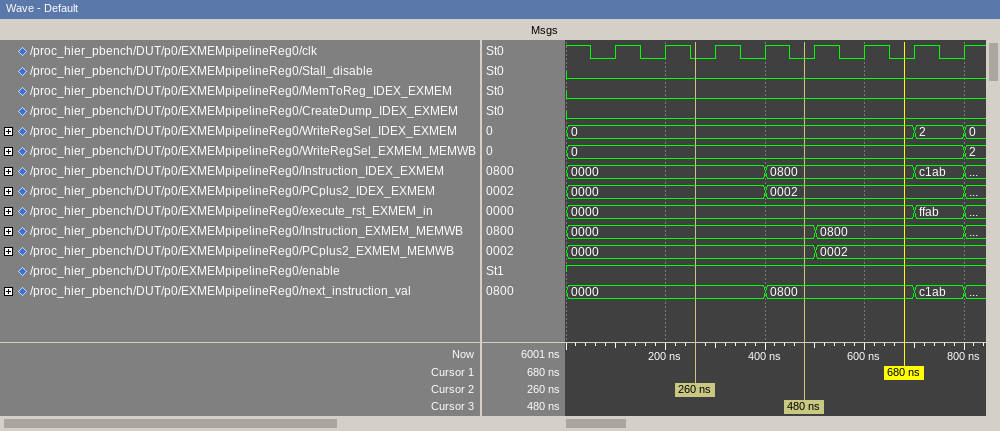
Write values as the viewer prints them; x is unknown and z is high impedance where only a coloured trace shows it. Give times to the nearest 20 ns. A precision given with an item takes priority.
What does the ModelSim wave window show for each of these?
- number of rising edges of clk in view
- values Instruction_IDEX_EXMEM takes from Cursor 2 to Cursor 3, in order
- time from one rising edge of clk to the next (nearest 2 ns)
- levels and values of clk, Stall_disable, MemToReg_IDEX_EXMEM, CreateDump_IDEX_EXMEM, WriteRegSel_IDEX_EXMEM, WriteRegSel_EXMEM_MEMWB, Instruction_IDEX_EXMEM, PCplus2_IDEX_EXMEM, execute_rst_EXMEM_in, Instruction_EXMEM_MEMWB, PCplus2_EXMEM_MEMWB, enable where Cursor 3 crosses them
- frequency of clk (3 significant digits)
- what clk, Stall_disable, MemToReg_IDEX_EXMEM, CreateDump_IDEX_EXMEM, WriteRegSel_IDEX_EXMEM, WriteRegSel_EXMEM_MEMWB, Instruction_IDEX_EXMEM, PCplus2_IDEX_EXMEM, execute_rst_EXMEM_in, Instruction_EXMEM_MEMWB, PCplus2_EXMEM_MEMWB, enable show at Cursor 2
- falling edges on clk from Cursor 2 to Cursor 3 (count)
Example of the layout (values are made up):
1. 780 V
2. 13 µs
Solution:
1. 8
2. 0000, 0800
3. 100 ns
4. clk=0, Stall_disable=0, MemToReg_IDEX_EXMEM=0, CreateDump_IDEX_EXMEM=0, WriteRegSel_IDEX_EXMEM=0, WriteRegSel_EXMEM_MEMWB=0, Instruction_IDEX_EXMEM=0800, PCplus2_IDEX_EXMEM=0002, execute_rst_EXMEM_in=0000, Instruction_EXMEM_MEMWB=0000, PCplus2_EXMEM_MEMWB=0000, enable=1
5. 10.0 MHz
6. clk=0, Stall_disable=0, MemToReg_IDEX_EXMEM=0, CreateDump_IDEX_EXMEM=0, WriteRegSel_IDEX_EXMEM=0, WriteRegSel_EXMEM_MEMWB=0, Instruction_IDEX_EXMEM=0000, PCplus2_IDEX_EXMEM=0000, execute_rst_EXMEM_in=0000, Instruction_EXMEM_MEMWB=0000, PCplus2_EXMEM_MEMWB=0000, enable=1
7. 2
